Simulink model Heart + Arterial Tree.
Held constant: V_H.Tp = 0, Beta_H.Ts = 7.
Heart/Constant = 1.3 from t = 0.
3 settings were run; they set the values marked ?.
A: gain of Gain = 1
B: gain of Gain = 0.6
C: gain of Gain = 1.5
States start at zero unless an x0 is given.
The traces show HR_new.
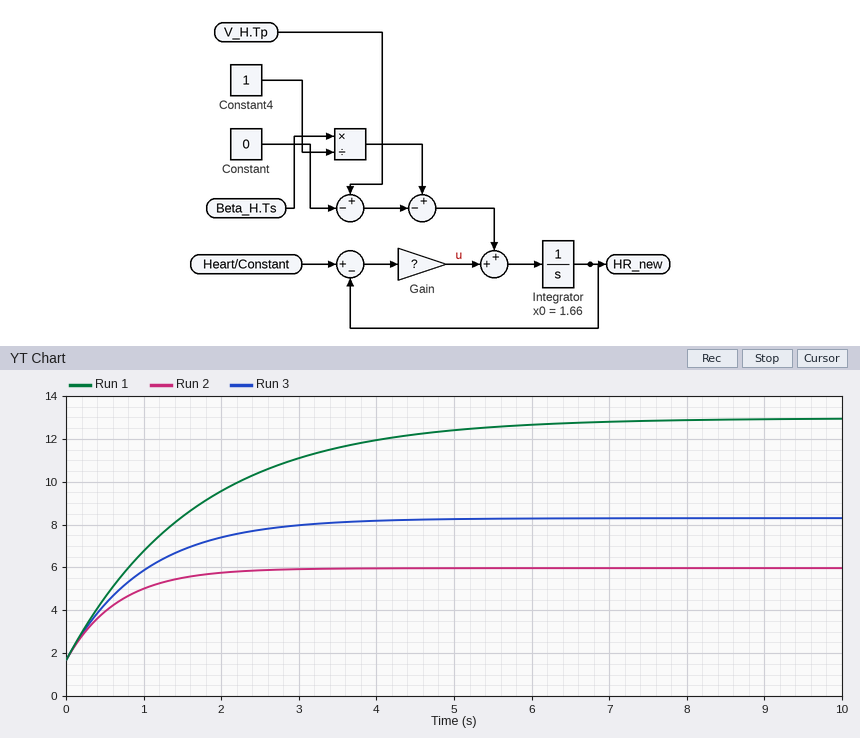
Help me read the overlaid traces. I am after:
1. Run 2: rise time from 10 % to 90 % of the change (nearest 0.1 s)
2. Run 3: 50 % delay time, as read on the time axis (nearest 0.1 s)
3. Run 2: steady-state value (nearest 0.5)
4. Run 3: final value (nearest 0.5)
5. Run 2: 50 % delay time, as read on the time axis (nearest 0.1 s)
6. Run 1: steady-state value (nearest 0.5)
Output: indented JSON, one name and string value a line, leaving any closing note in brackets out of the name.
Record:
{
  "Run 2: rise time from 10 % to 90 % of the change": "1.5 s",
  "Run 3: 50 % delay time, as read on the time axis": "0.7 s",
  "Run 2: steady-state value": "6.0",
  "Run 3: final value": "8.5",
  "Run 2: 50 % delay time, as read on the time axis": "0.5 s",
  "Run 1: steady-state value": "13.0"
}
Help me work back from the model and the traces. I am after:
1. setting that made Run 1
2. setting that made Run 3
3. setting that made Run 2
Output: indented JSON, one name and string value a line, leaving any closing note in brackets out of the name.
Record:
{
  "setting that made Run 1": "B",
  "setting that made Run 3": "A",
  "setting that made Run 2": "C"
}
